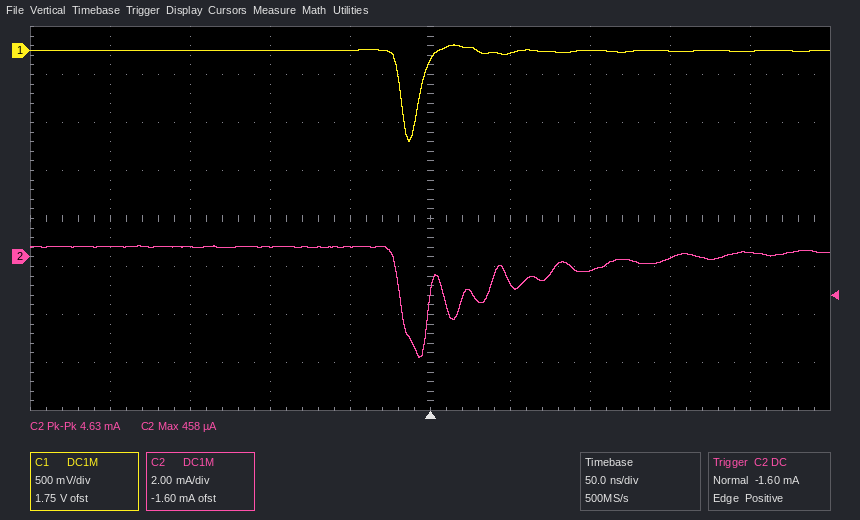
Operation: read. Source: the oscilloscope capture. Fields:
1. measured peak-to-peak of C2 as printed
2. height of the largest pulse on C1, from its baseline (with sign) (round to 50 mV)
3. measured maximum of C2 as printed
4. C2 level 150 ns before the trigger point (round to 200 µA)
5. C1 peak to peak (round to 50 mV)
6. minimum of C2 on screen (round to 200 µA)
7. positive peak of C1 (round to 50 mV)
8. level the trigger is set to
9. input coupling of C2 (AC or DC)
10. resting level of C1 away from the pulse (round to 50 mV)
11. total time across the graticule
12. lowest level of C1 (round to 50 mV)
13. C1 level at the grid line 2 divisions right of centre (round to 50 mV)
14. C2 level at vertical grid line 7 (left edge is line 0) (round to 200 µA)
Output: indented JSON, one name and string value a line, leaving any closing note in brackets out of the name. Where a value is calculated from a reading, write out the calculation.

{
  "measured peak-to-peak of C2 as printed": "4.63 mA",
  "height of the largest pulse on C1, from its baseline (with sign)": "-950 mV − (0 mV) = -950 mV",
  "measured maximum of C2 as printed": "458 µA",
  "C2 level 150 ns before the trigger point": "400 µA",
  "C1 peak to peak": "50 mV − (-950 mV) = 1.00 V",
  "minimum of C2 on screen": "-4.2 mA",
  "positive peak of C1": "50 mV",
  "level the trigger is set to": "-1.60 mA",
  "input coupling of C2": "DC",
  "resting level of C1 away from the pulse": "0 mV",
  "total time across the graticule": "500 ns",
  "lowest level of C1": "-950 mV",
  "C1 level at the grid line 2 divisions right of centre": "0 mV",
  "C2 level at vertical grid line 7 (left edge is line 0)": "-600 µA"
}
